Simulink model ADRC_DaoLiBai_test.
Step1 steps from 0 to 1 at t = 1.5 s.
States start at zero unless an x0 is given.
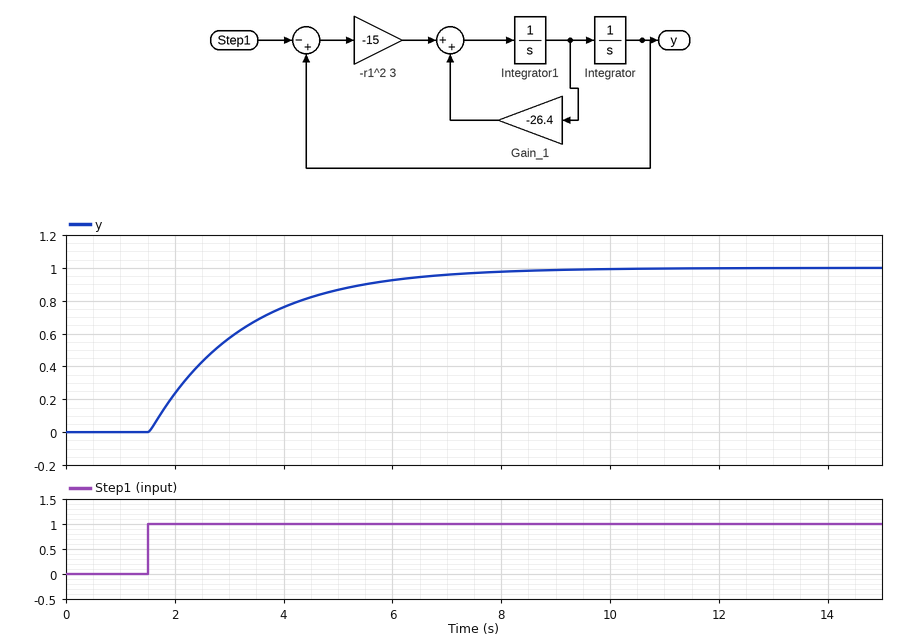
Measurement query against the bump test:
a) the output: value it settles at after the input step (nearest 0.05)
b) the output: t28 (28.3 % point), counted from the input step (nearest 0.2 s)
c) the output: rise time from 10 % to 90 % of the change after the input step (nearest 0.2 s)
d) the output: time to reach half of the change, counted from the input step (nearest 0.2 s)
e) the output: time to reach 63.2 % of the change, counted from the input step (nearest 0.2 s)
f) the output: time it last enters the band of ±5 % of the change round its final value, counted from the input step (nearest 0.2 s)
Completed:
1.00
0.6 s
3.8 s
1.2 s
1.8 s
5.2 s
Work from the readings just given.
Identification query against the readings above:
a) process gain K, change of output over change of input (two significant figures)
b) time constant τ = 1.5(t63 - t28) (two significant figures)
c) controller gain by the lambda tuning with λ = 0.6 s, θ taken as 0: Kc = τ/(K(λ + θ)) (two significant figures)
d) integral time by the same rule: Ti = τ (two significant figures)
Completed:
1.0
1.8 s
3.0
1.8 s
